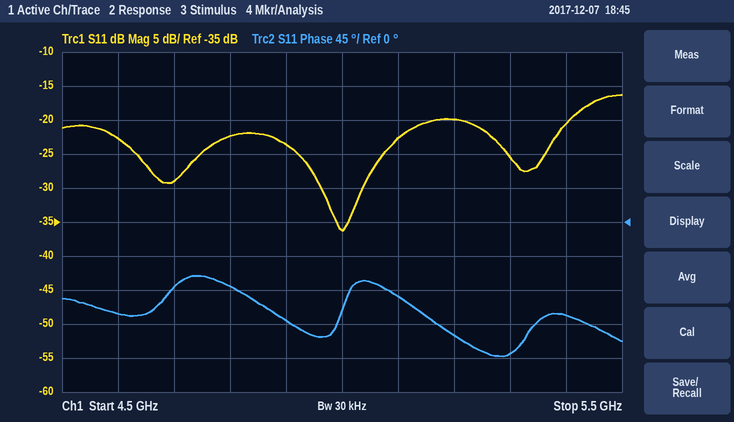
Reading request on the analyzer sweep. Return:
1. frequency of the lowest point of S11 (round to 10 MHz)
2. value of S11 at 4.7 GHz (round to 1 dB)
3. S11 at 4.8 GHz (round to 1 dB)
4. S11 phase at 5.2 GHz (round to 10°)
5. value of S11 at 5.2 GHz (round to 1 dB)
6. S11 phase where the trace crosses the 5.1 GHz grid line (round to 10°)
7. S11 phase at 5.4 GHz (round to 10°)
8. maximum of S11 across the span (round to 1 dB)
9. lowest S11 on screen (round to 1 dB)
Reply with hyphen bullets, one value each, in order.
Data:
- 5.00 GHz
- -29 dB
- -22 dB
- -150°
- -20 dB
- -100°
- -120°
- -16 dB
- -36 dB
